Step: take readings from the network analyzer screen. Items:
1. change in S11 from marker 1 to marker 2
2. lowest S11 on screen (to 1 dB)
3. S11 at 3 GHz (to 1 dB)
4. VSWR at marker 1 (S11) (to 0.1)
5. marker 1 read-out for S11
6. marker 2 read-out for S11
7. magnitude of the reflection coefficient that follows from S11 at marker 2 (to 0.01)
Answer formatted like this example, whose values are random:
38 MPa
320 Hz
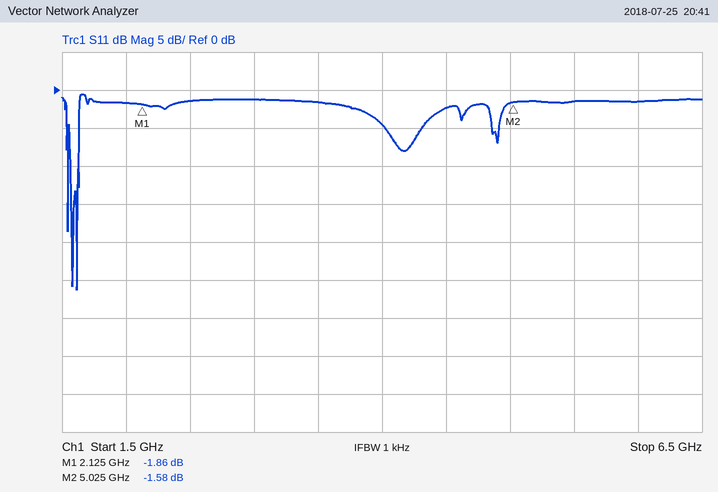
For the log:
0.28 dB
-26 dB
-1 dB
9.4
-1.86 dB
-1.58 dB
0.83
